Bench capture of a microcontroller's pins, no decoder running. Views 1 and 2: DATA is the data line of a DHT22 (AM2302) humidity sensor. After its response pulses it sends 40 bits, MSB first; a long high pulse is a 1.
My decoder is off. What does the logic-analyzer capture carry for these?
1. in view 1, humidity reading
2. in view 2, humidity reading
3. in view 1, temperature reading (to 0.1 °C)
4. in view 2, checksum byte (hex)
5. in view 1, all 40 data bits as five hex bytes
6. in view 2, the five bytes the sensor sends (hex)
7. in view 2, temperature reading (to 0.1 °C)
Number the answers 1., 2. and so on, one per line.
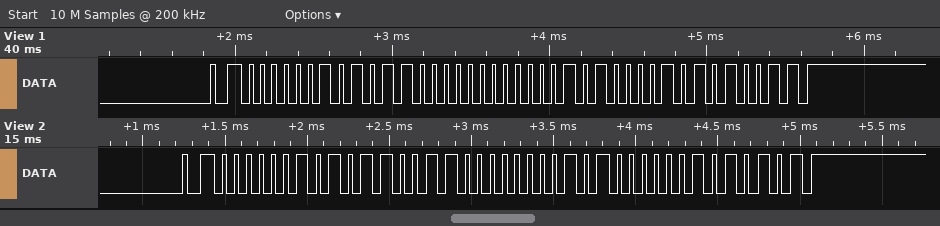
1. 68.8 %
2. 69.1 %
3. 16.1 °C
4. 0x55
5. 02 B0 00 A1 53
6. 02 B3 00 A0 55
7. 16.0 °C
